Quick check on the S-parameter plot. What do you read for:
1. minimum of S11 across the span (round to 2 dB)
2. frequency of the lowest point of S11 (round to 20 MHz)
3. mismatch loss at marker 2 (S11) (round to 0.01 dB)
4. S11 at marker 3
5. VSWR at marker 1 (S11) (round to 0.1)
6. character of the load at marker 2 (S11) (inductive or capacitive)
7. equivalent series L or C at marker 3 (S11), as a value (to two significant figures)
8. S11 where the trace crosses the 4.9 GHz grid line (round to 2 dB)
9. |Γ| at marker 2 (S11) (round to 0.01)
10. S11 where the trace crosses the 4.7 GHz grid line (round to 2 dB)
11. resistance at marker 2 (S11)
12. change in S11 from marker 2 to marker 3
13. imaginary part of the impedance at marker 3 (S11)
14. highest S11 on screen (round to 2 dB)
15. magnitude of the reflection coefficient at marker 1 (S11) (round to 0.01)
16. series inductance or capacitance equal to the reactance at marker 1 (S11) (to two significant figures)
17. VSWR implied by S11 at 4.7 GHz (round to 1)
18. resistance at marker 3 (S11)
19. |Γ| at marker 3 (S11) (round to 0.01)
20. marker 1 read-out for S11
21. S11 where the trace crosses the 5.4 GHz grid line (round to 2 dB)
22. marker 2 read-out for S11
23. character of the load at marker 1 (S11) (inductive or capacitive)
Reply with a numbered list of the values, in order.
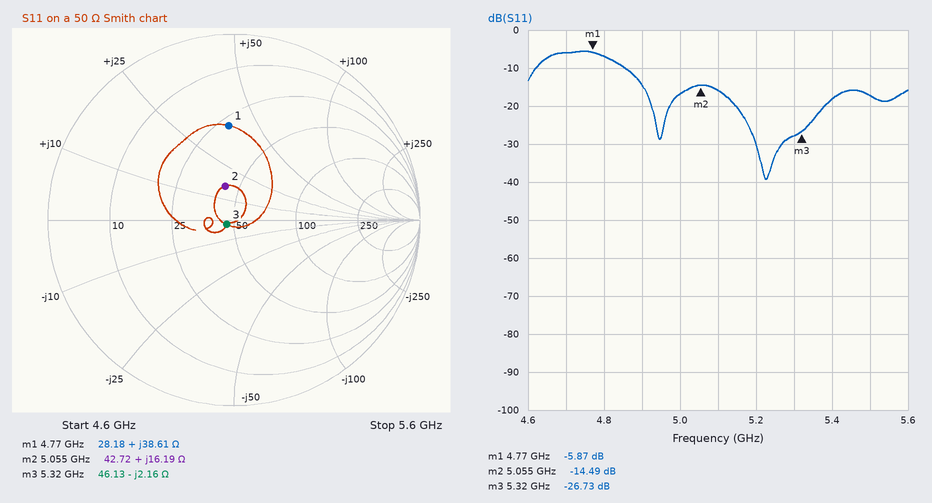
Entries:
1. -40 dB
2. 5.22 GHz
3. 0.16 dB
4. -26.73 dB
5. 3.1
6. inductive
7. 14 pF
8. -14 dB
9. 0.19
10. -6 dB
11. 42.72 Ω
12. -12.24 dB
13. -2.16 Ω
14. -6 dB
15. 0.51
16. 1.3 nH
17. 3
18. 46.13 Ω
19. 0.05
20. -5.87 dB
21. -18 dB
22. -14.49 dB
23. inductive
